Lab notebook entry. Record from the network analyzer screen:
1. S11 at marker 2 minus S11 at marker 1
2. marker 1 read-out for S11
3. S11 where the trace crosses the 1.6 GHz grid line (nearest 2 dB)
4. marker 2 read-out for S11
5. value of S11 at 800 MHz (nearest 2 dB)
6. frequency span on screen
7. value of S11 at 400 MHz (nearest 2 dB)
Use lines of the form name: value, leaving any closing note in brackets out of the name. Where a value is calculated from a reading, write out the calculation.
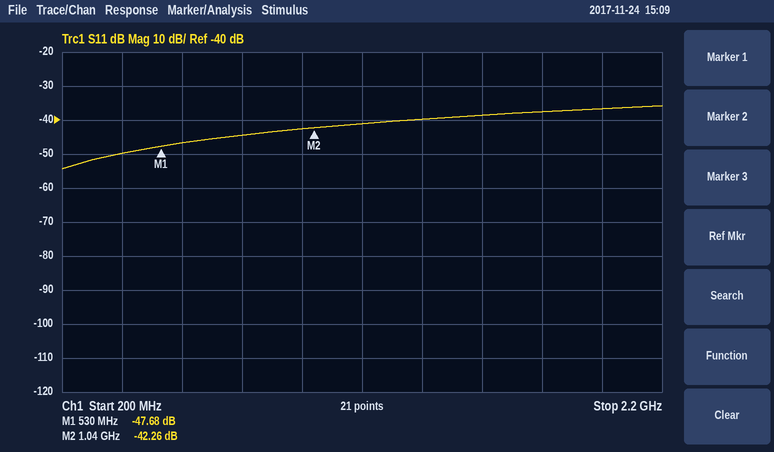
S11 at marker 2 minus S11 at marker 1: -42.26 − (-47.68) = 5.42 dB
marker 1 read-out for S11: -47.68 dB
S11 where the trace crosses the 1.6 GHz grid line: -38 dB
marker 2 read-out for S11: -42.26 dB
value of S11 at 800 MHz: -44 dB
frequency span on screen: 2 GHz
value of S11 at 400 MHz: -50 dB
